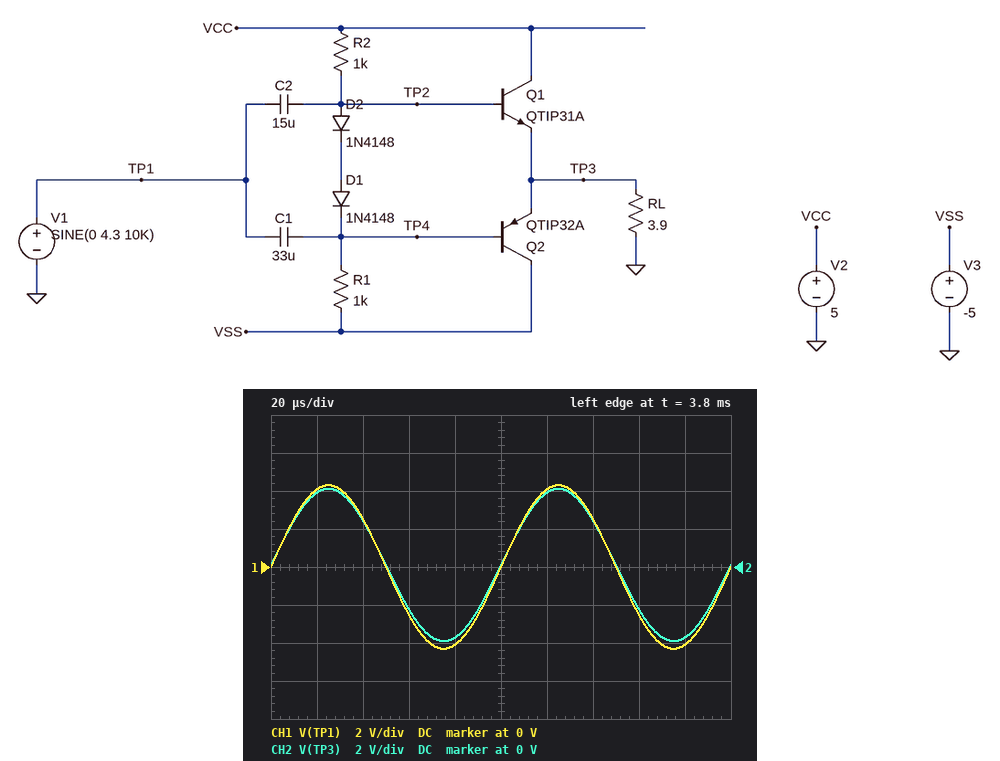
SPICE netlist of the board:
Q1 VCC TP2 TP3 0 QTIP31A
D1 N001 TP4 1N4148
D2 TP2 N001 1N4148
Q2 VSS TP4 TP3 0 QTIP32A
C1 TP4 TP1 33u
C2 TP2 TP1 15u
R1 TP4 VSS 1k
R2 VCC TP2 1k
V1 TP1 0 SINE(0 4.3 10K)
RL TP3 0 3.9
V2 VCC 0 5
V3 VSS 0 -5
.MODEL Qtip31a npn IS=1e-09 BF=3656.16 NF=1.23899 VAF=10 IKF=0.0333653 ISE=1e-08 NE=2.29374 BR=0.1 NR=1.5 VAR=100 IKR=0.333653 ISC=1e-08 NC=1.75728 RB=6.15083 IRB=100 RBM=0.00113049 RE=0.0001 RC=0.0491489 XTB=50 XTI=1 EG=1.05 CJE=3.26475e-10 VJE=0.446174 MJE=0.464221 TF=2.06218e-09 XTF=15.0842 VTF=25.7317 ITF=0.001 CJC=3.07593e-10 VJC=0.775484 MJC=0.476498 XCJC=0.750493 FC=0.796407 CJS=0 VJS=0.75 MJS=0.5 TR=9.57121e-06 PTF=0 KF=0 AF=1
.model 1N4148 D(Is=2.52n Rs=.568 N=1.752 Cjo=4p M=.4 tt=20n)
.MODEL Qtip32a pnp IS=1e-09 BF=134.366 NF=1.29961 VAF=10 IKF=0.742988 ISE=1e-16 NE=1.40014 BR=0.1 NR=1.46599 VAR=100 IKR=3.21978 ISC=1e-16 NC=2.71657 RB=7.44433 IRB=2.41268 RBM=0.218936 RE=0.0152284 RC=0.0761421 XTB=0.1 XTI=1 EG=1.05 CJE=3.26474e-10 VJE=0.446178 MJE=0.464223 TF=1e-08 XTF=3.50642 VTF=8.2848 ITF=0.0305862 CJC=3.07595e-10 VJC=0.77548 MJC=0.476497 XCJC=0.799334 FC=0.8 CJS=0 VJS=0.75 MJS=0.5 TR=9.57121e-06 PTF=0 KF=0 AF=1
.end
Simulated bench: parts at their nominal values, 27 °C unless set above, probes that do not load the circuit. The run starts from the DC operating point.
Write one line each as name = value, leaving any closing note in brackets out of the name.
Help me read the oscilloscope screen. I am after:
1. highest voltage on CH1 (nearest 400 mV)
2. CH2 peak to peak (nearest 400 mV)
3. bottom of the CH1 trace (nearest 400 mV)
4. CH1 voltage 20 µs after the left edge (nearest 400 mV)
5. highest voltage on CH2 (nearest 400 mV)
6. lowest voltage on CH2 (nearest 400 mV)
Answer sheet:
highest voltage on CH1 = 4.4 V
CH2 peak to peak = 8.0 V
bottom of the CH1 trace = -4.4 V
CH1 voltage 20 µs after the left edge = 4.0 V
highest voltage on CH2 = 4.0 V
lowest voltage on CH2 = -4.0 V
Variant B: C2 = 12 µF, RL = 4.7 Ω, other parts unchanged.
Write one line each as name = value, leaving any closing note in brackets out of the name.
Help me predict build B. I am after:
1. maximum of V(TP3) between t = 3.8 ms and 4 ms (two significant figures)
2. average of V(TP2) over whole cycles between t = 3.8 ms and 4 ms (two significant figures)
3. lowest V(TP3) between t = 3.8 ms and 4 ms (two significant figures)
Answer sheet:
maximum of V(TP3) between t = 3.8 ms and 4 ms = 4.2 V
average of V(TP2) over whole cycles between t = 3.8 ms and 4 ms = 720 mV
lowest V(TP3) between t = 3.8 ms and 4 ms = -4.0 V
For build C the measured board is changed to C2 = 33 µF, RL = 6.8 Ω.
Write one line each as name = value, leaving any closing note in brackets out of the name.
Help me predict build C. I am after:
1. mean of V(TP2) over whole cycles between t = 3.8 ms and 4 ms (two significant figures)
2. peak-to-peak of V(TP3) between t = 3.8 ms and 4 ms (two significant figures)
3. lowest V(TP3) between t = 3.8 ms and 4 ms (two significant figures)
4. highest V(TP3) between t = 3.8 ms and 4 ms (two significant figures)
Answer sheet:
mean of V(TP2) over whole cycles between t = 3.8 ms and 4 ms = 750 mV
peak-to-peak of V(TP3) between t = 3.8 ms and 4 ms = 8.3 V
lowest V(TP3) between t = 3.8 ms and 4 ms = -4.0 V
highest V(TP3) between t = 3.8 ms and 4 ms = 4.3 V
